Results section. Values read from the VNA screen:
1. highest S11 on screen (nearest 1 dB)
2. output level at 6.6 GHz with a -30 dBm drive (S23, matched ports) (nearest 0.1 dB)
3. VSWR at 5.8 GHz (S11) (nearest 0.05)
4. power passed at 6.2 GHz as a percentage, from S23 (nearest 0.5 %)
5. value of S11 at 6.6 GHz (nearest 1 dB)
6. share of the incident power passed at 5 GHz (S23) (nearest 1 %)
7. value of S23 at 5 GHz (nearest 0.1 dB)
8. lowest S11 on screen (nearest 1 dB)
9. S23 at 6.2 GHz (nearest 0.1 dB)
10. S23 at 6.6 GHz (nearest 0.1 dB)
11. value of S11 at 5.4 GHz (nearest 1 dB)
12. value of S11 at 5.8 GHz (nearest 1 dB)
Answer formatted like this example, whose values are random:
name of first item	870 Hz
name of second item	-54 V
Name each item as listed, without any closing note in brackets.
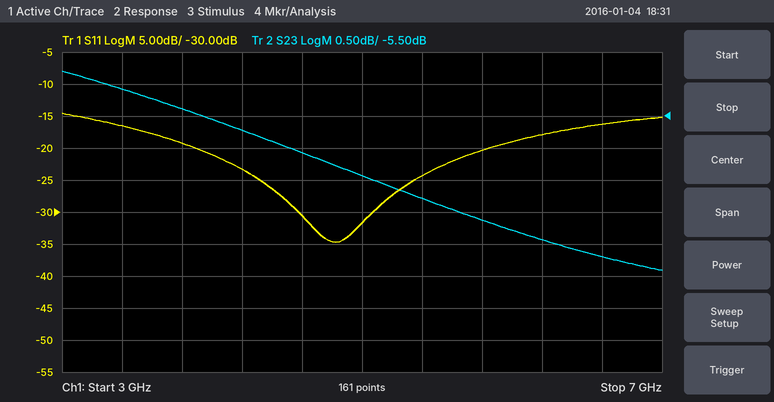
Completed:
highest S11 on screen	-15 dB
output level at 6.6 GHz with a -30 dBm drive (S23, matched ports)	-37.7 dBm
VSWR at 5.8 GHz (S11)	1.20
power passed at 6.2 GHz as a percentage, from S23	18.0 %
value of S11 at 6.6 GHz	-16 dB
share of the incident power passed at 5 GHz (S23)	23 %
value of S23 at 5 GHz	-6.4 dB
lowest S11 on screen	-35 dB
S23 at 6.2 GHz	-7.4 dB
S23 at 6.6 GHz	-7.7 dB
value of S11 at 5.4 GHz	-24 dB
value of S11 at 5.8 GHz	-20 dB
